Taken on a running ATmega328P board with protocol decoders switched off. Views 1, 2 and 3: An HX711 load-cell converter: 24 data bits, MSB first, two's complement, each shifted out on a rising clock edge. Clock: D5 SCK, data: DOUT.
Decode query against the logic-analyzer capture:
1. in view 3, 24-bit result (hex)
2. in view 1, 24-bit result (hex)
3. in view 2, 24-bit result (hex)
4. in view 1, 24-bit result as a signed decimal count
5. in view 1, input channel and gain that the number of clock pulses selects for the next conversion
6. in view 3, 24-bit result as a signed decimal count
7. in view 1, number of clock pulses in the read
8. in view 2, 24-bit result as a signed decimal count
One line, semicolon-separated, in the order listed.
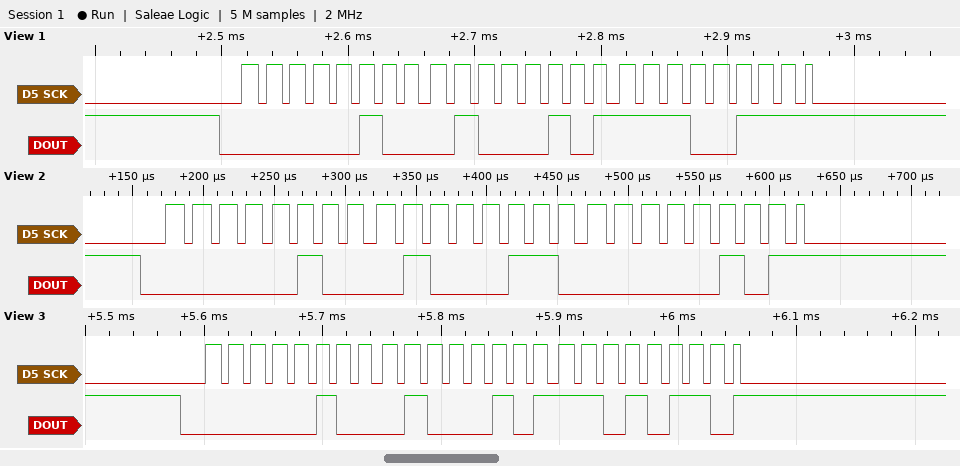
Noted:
0x0445D6; 0x0445E7; 0x044605; 280039; channel A, gain 128; 280022; 25; 280069
